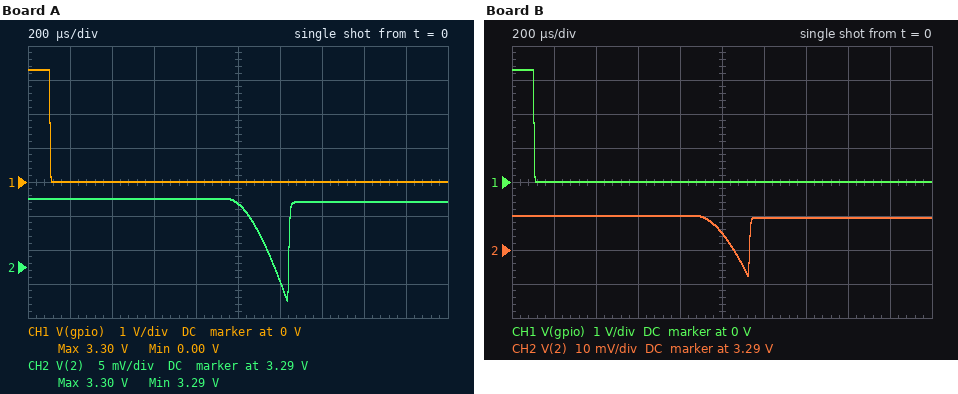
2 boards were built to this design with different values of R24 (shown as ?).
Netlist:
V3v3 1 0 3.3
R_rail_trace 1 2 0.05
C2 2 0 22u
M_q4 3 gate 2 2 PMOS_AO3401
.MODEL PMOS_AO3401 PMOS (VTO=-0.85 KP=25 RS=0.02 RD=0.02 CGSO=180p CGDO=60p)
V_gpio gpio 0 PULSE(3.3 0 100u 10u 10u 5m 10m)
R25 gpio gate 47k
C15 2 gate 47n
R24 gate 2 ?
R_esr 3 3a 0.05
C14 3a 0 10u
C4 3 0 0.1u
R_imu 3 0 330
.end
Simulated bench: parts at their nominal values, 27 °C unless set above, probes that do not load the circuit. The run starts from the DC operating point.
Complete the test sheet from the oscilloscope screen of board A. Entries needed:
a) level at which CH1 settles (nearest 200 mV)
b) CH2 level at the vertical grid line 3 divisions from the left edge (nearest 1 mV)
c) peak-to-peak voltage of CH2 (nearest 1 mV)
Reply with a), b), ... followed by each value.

a) 0 V
b) 3.300 V
c) 15 mV
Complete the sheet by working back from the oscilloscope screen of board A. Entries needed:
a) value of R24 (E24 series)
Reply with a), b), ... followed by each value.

a) 39 kΩ
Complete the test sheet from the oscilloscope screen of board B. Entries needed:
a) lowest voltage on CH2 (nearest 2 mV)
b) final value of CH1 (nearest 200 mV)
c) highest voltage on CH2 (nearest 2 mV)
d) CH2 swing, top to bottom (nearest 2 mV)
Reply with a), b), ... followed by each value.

a) 3.282 V
b) 0 V
c) 3.300 V
d) 18 mV
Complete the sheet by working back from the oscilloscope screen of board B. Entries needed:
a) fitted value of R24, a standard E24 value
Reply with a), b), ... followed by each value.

a) 56 kΩ
